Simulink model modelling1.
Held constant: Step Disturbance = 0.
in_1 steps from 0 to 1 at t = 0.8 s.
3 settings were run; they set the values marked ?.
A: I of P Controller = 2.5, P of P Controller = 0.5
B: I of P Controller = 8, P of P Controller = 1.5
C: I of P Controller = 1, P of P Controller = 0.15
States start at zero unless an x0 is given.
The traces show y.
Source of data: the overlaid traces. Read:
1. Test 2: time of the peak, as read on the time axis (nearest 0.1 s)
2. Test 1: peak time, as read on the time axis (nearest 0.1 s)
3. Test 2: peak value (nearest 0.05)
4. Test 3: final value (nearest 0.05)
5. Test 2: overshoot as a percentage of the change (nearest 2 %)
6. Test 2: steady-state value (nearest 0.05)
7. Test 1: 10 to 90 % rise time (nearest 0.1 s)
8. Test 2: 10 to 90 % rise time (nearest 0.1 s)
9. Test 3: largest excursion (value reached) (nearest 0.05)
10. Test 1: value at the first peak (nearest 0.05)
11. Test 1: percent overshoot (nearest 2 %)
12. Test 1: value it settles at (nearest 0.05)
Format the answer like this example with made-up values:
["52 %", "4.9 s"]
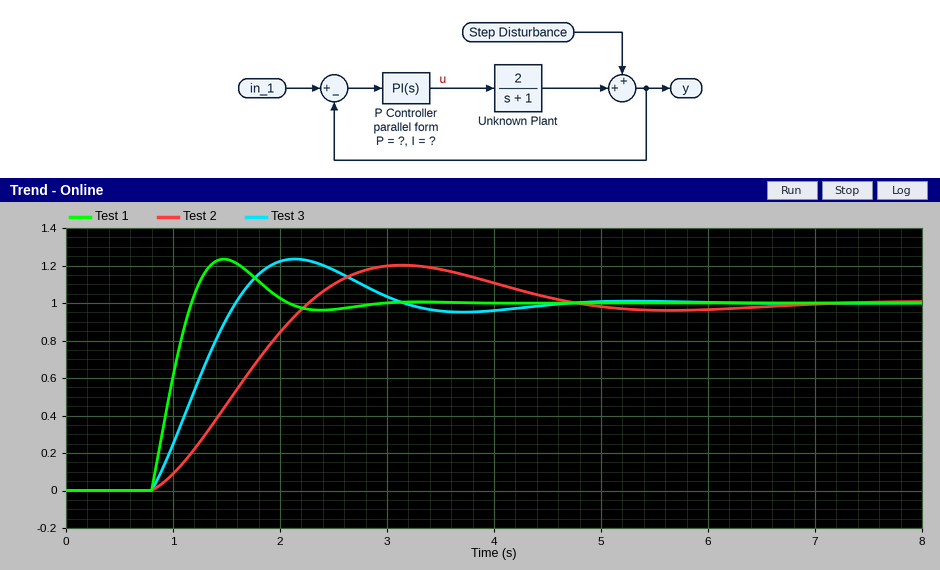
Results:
["3.1 s", "1.5 s", "1.20", "1.00", "20 %", "1.00", "0.3 s", "1.1 s", "1.25", "1.25", "24 %", "1.00"]
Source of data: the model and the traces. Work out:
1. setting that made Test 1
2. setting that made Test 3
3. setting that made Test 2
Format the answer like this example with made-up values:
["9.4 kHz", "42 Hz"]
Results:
["B", "A", "C"]
